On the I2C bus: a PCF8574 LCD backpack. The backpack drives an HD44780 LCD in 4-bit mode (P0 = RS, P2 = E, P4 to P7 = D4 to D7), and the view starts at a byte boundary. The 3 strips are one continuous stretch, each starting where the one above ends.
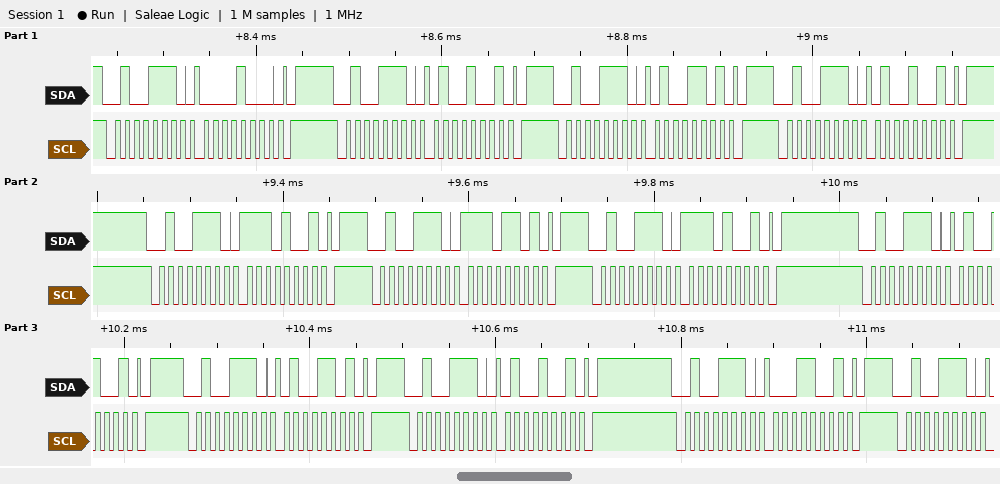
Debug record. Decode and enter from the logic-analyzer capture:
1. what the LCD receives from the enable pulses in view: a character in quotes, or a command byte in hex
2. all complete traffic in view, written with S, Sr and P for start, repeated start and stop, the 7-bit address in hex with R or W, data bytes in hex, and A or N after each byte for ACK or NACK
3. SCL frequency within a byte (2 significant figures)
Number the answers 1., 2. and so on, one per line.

1. 'N'
2. S 27W A 08 A P S 27W A 49 A P S 27W A 4D A P S 27W A 49 A P S 27W A E9 A P S 27W A ED A P S 27W A E9 A P S 27W A 49 A P S 27W A 4D A P S 27W A 49 A P S 27W A 19 A P S 27W A
3. 100 kHz
